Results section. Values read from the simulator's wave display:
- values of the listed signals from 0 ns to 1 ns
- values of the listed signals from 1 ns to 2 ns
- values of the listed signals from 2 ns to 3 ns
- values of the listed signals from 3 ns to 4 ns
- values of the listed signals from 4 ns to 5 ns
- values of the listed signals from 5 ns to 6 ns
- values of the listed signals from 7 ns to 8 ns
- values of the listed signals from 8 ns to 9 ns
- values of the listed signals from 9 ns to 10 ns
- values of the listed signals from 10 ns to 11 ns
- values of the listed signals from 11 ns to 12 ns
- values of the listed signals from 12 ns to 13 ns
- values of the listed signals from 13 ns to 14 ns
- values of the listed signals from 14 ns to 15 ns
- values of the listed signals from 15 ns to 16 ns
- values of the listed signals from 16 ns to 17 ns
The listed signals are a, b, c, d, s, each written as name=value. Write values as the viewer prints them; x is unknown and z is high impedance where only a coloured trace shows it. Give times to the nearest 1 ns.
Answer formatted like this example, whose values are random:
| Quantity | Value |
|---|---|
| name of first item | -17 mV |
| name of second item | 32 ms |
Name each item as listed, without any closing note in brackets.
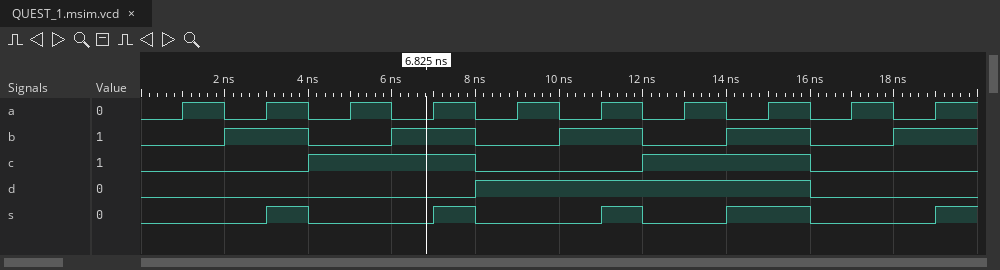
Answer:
| Quantity | Value |
|---|---|
| values of the listed signals from 0 ns to 1 ns | a=0, b=0, c=0, d=0, s=0 |
| values of the listed signals from 1 ns to 2 ns | a=1, b=0, c=0, d=0, s=0 |
| values of the listed signals from 2 ns to 3 ns | a=0, b=1, c=0, d=0, s=0 |
| values of the listed signals from 3 ns to 4 ns | a=1, b=1, c=0, d=0, s=1 |
| values of the listed signals from 4 ns to 5 ns | a=0, b=0, c=1, d=0, s=0 |
| values of the listed signals from 5 ns to 6 ns | a=1, b=0, c=1, d=0, s=0 |
| values of the listed signals from 7 ns to 8 ns | a=1, b=1, c=1, d=0, s=1 |
| values of the listed signals from 8 ns to 9 ns | a=0, b=0, c=0, d=1, s=0 |
| values of the listed signals from 9 ns to 10 ns | a=1, b=0, c=0, d=1, s=0 |
| values of the listed signals from 10 ns to 11 ns | a=0, b=1, c=0, d=1, s=0 |
| values of the listed signals from 11 ns to 12 ns | a=1, b=1, c=0, d=1, s=1 |
| values of the listed signals from 12 ns to 13 ns | a=0, b=0, c=1, d=1, s=0 |
| values of the listed signals from 13 ns to 14 ns | a=1, b=0, c=1, d=1, s=0 |
| values of the listed signals from 14 ns to 15 ns | a=0, b=1, c=1, d=1, s=1 |
| values of the listed signals from 15 ns to 16 ns | a=1, b=1, c=1, d=1, s=1 |
| values of the listed signals from 16 ns to 17 ns | a=0, b=0, c=0, d=0, s=0 |
